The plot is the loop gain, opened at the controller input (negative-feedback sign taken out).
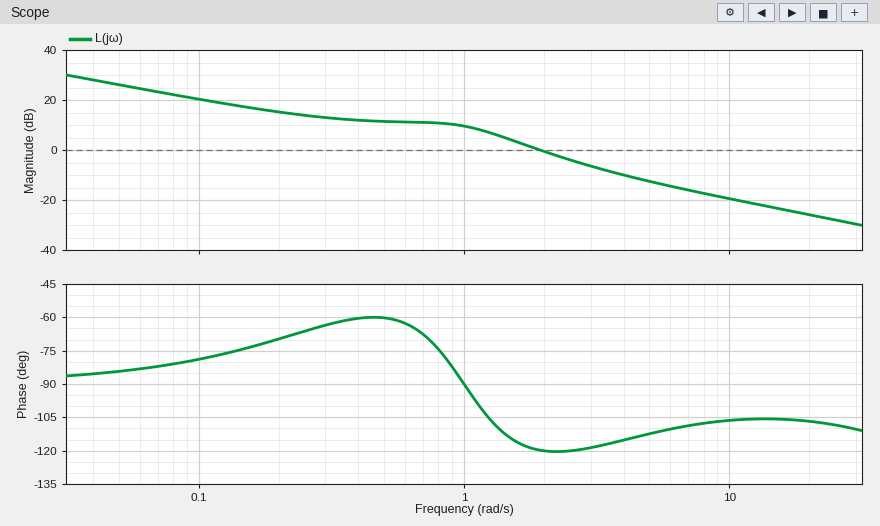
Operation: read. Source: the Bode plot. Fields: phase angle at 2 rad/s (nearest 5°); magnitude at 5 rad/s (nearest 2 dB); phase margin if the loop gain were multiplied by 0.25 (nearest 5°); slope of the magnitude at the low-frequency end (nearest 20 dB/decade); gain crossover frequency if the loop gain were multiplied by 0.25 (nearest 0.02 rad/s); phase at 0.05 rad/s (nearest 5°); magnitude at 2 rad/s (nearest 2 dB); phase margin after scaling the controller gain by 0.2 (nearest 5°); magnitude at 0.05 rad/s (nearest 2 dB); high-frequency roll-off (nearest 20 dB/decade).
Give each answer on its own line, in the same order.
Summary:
-120°
-12 dB
120°
-20 dB/decade
0.38 rad/s
-85°
0 dB
115°
26 dB
-20 dB/decade
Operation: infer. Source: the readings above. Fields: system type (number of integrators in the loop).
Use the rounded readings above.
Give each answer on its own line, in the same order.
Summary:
1
